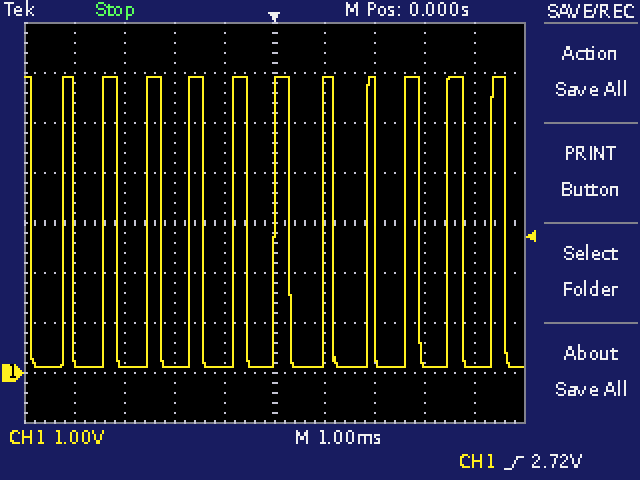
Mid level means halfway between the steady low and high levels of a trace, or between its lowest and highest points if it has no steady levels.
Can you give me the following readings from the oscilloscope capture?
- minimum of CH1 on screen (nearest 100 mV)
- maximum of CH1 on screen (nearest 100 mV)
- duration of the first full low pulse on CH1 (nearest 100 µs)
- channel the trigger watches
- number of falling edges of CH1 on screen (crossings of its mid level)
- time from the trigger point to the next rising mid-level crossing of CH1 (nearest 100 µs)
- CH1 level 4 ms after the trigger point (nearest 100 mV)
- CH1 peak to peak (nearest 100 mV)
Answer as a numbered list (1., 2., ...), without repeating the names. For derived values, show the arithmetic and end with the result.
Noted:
1. 100 mV
2. 5.9 V
3. 600 µs
4. CH1
5. 12
6. 1.0 ms
7. 100 mV
8. 5.9 V − (100 mV) = 5.8 V
